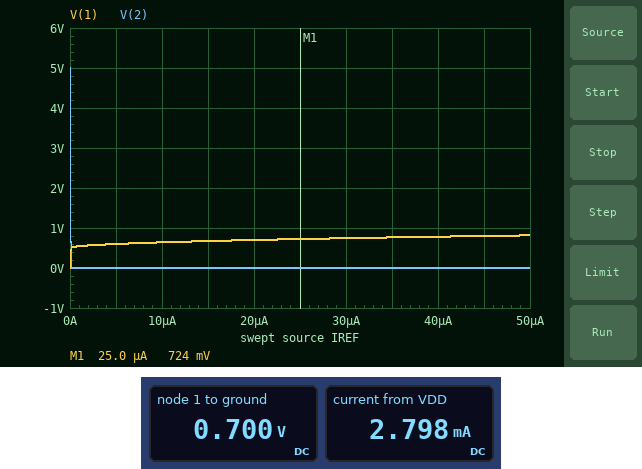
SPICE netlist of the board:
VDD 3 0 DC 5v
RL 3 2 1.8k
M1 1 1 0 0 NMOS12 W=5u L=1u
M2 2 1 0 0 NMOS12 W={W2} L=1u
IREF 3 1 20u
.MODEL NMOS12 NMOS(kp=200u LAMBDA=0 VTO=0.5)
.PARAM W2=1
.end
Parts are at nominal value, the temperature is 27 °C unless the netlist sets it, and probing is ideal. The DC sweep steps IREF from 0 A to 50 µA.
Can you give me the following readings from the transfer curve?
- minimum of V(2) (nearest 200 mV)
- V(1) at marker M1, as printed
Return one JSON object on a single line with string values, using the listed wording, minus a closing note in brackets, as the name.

{"minimum of V(2)": "0 V", "V(1) at marker M1, as printed": "724 mV"}
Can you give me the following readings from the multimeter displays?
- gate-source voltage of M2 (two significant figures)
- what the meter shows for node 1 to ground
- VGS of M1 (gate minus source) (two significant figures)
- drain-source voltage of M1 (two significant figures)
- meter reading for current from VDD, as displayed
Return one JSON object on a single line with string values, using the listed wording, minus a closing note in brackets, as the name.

{"gate-source voltage of M2": "700 mV", "what the meter shows for node 1 to ground": "0.700 V", "VGS of M1 (gate minus source)": "700 mV", "drain-source voltage of M1": "700 mV", "meter reading for current from VDD, as displayed": "2.798 mA"}
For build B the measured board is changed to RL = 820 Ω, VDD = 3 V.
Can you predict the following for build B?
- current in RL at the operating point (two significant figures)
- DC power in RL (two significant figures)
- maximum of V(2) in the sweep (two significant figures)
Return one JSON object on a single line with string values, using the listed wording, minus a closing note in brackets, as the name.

{"current in RL at the operating point": "3.7 mA", "DC power in RL": "11 mW", "maximum of V(2) in the sweep": "3.0 V"}
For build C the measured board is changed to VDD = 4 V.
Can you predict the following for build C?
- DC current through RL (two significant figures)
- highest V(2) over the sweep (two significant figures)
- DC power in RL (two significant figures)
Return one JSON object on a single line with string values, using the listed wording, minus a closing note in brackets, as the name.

{"DC current through RL": "2.2 mA", "highest V(2) over the sweep": "4.0 V", "DC power in RL": "8.9 mW"}
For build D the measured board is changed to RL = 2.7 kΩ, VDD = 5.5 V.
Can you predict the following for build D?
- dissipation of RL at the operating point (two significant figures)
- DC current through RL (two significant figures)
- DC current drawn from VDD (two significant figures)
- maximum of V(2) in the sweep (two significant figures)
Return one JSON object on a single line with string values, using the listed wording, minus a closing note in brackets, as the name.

{"dissipation of RL at the operating point": "11 mW", "DC current through RL": "2.0 mA", "DC current drawn from VDD": "2.1 mA", "maximum of V(2) in the sweep": "5.5 V"}
